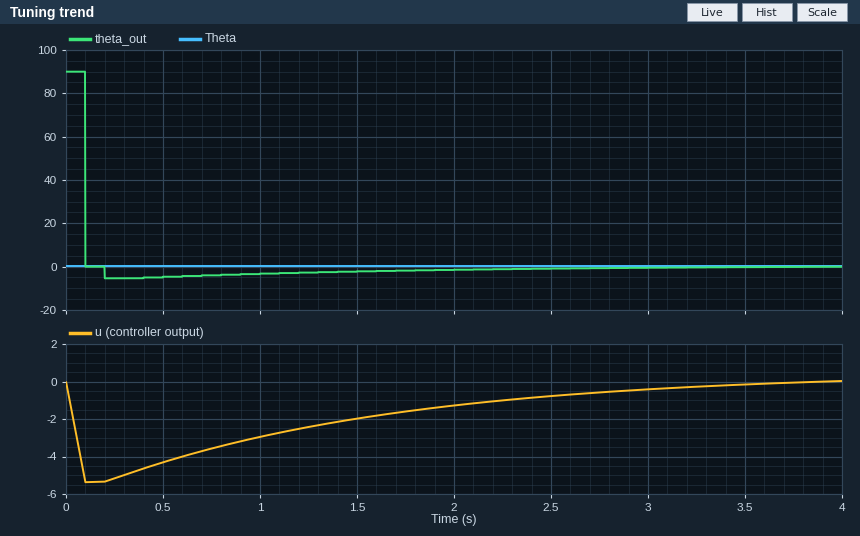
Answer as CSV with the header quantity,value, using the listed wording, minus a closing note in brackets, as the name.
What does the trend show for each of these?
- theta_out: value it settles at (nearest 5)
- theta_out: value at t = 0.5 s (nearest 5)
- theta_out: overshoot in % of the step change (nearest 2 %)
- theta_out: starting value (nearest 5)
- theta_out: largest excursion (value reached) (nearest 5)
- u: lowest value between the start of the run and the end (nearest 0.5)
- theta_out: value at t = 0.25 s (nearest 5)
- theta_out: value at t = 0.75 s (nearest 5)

quantity,value
theta_out: value it settles at,0
theta_out: value at t = 0.5 s,-5
theta_out: overshoot in % of the step change,6 %
theta_out: starting value,90
theta_out: largest excursion (value reached),-5
u: lowest value between the start of the run and the end,-5.5
theta_out: value at t = 0.25 s,-5
theta_out: value at t = 0.75 s,-5
